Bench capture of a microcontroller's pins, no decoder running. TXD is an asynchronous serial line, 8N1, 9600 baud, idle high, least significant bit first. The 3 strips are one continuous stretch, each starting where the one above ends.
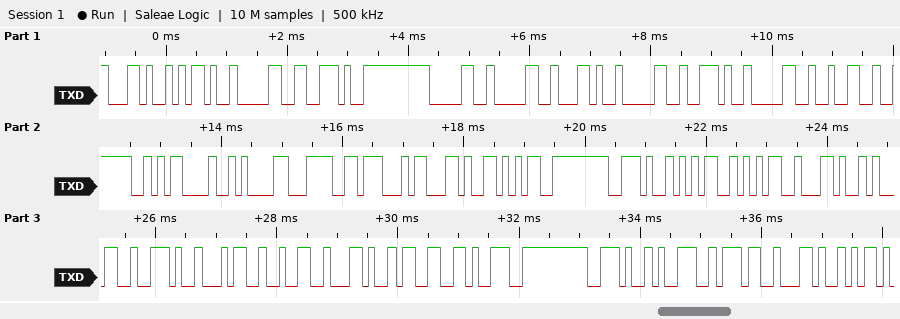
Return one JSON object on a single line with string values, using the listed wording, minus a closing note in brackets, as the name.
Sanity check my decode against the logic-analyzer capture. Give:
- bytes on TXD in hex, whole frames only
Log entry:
{"bytes on TXD in hex, whole frames only": "2C 2D 30 2E 30 30 2C 30 2E 30 32 3E 0D 0A 3C 47 2C 35 2E 35 35 2C 31 2E 34 32 2C 33 39 2E 39 37 2C"}
